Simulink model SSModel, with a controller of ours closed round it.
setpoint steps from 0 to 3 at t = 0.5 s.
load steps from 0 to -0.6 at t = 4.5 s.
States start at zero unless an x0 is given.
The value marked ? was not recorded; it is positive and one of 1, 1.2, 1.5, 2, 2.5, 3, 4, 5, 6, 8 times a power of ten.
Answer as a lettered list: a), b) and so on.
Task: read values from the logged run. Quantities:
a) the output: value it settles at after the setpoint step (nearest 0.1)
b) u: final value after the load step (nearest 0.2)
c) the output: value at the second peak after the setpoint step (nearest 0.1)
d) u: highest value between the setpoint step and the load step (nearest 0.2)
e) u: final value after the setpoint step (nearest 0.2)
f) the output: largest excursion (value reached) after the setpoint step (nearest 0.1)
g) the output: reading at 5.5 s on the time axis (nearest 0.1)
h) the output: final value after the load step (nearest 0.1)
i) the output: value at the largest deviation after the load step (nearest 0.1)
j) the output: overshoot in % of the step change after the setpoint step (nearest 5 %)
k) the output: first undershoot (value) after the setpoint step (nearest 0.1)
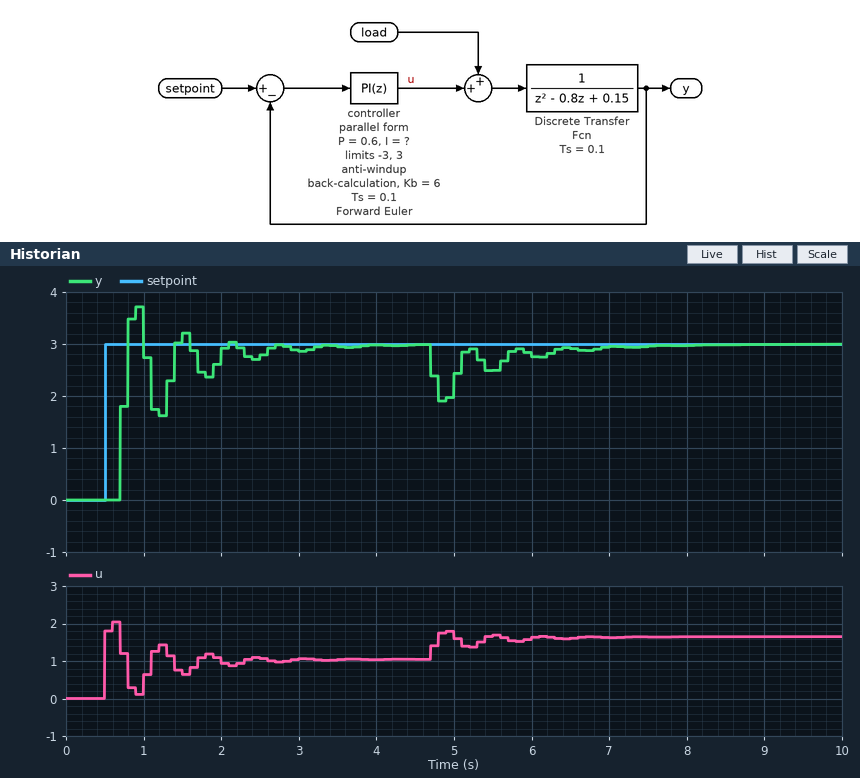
a) 3.0
b) 1.6
c) 3.2
d) 2.0
e) 1.0
f) 3.7
g) 2.5
h) 3.0
i) 1.9
j) 25 %
k) 1.6
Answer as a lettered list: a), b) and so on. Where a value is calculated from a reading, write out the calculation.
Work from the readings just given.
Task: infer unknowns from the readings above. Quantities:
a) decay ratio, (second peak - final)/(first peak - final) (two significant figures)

a) (3.2 - 3) / (3.7 - 3) = 0.29
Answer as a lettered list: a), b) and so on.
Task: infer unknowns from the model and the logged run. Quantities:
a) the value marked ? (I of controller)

a) 0.8
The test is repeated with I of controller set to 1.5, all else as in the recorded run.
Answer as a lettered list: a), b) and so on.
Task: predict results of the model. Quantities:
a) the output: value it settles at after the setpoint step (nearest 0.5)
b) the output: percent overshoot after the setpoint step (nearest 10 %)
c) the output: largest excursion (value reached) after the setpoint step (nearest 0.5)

a) 3.0
b) 40 %
c) 4.5
